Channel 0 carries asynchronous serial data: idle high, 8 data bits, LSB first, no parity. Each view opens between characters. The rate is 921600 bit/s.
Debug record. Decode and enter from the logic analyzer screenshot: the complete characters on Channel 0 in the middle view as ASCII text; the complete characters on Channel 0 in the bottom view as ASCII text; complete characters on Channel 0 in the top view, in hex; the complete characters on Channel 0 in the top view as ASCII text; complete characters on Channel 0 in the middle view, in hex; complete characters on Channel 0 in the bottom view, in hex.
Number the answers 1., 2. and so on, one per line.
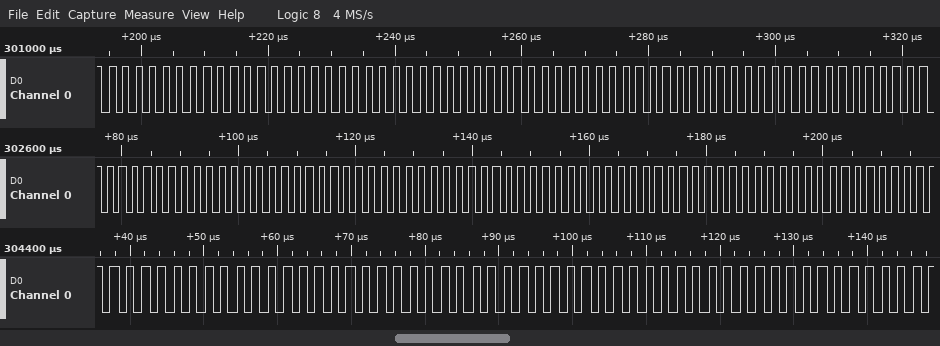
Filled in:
1. "UUUUUUUUUUUUU"
2. "UUUUUUUUUU"
3. 55, 55, 55, 55, 55, 55, 55, 55, 55, 55, 55, 55
4. "UUUUUUUUUUUU"
5. 55, 55, 55, 55, 55, 55, 55, 55, 55, 55, 55, 55, 55
6. 55, 55, 55, 55, 55, 55, 55, 55, 55, 55
